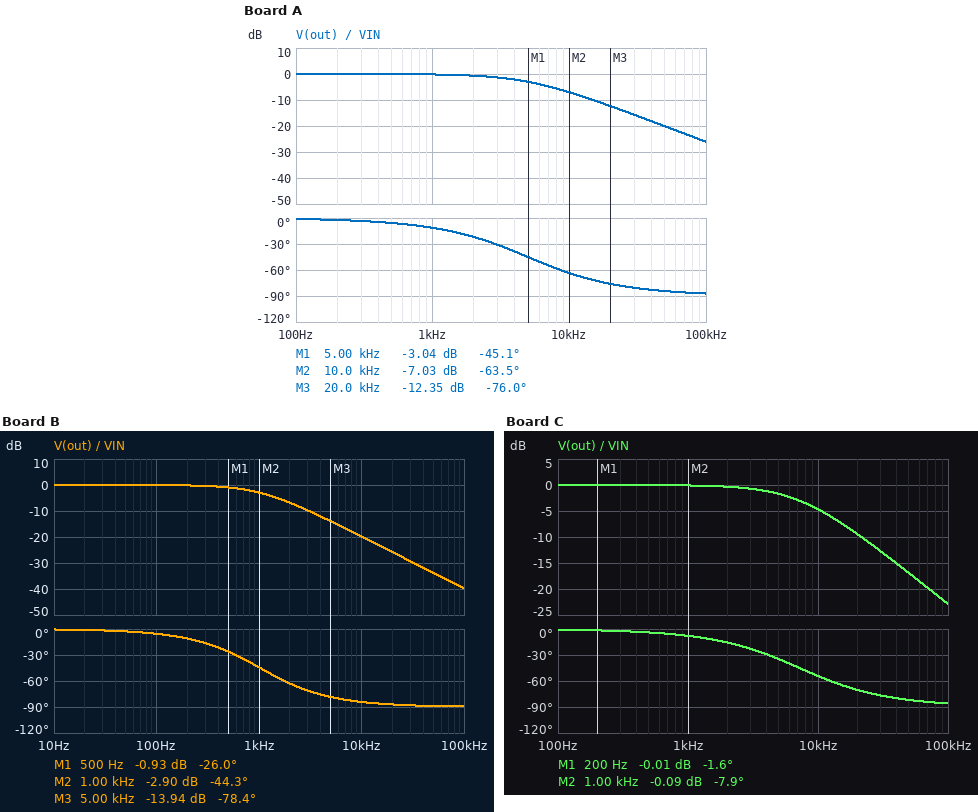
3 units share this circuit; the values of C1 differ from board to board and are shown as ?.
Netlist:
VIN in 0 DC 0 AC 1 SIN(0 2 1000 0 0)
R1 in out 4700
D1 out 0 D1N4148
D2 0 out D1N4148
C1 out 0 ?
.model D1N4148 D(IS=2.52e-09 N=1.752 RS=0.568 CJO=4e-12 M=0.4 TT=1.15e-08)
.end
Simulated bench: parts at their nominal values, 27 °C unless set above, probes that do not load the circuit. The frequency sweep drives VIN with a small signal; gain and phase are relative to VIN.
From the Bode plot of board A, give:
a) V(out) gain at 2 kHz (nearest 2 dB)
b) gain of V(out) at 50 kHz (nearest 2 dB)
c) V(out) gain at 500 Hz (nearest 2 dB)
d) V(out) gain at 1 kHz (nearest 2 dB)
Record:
0 dB
-20 dB
0 dB
0 dB
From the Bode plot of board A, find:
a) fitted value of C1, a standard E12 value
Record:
6.8 nF
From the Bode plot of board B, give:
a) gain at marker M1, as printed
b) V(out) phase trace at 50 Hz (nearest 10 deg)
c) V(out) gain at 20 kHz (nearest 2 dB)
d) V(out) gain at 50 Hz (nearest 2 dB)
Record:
-0.93 dB
0 deg
-26 dB
0 dB
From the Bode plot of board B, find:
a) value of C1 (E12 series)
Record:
33 nF
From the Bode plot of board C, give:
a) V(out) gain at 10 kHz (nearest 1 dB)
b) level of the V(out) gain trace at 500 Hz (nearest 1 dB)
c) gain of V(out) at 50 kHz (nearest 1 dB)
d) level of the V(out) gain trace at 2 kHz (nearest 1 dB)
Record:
-5 dB
0 dB
-17 dB
0 dB
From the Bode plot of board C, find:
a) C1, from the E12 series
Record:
4.7 nF
